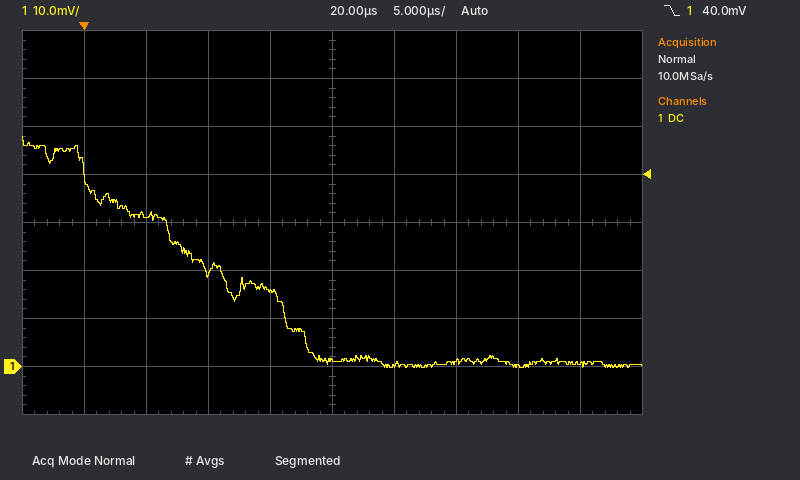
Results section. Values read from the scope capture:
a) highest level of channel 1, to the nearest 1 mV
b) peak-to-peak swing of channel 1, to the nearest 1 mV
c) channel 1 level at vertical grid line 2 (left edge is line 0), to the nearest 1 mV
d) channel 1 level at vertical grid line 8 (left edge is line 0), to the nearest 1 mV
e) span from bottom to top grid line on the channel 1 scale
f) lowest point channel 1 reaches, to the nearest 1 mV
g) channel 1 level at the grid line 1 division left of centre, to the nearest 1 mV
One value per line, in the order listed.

48 mV
48 mV
31 mV
0 mV
80 mV
0 mV
16 mV
